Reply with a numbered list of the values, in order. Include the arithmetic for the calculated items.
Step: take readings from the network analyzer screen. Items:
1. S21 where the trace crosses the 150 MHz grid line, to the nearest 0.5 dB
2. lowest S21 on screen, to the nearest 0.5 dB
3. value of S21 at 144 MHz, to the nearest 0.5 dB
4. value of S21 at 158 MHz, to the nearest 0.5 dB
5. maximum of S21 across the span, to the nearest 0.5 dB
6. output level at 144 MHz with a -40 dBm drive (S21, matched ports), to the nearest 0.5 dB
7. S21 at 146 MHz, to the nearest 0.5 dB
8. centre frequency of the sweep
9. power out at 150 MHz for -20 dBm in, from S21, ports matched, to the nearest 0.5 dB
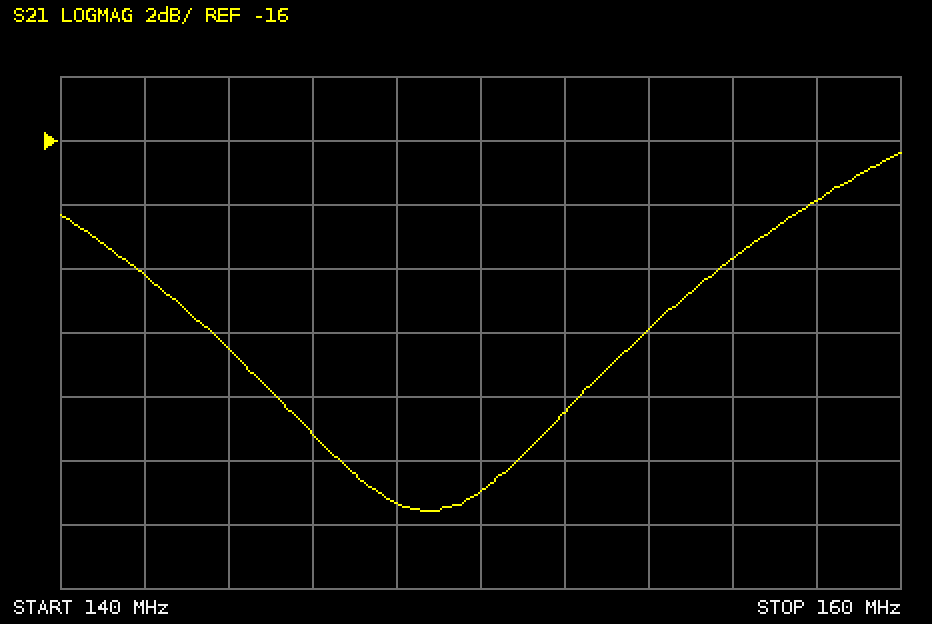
1. -27.0 dB
2. -27.5 dB
3. -22.5 dB
4. -18.0 dB
5. -16.5 dB
6. -40 dBm + (-22.5 dB) = -62.5 dBm
7. -25.0 dB
8. 150 MHz
9. -20 dBm + (-27.0 dB) = -47.0 dBm
